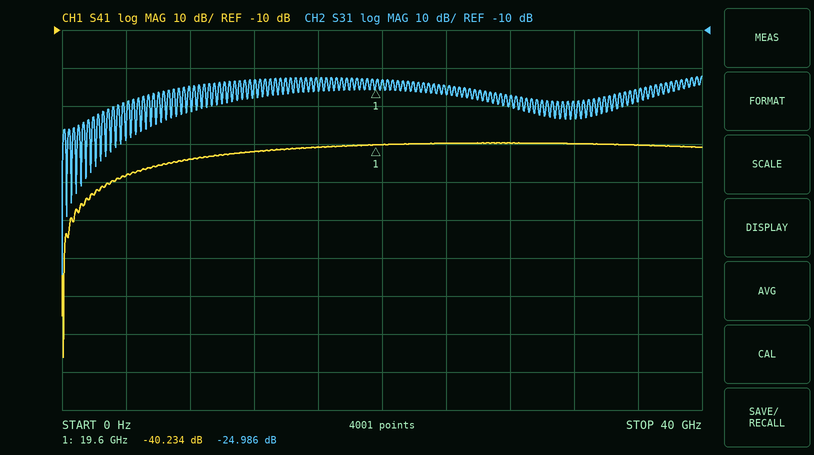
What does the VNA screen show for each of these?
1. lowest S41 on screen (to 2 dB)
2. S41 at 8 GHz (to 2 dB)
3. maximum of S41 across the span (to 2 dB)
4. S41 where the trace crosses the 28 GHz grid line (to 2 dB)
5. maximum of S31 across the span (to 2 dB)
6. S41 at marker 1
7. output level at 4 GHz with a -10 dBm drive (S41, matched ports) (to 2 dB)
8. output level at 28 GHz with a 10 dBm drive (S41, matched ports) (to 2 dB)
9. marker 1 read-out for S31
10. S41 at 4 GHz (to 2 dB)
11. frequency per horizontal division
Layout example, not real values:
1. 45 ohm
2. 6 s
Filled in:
1. -96 dB
2. -44 dB
3. -40 dB
4. -40 dB
5. -22 dB
6. -40.234 dB
7. -58 dBm
8. -30 dBm
9. -24.986 dB
10. -48 dB
11. 4 GHz
